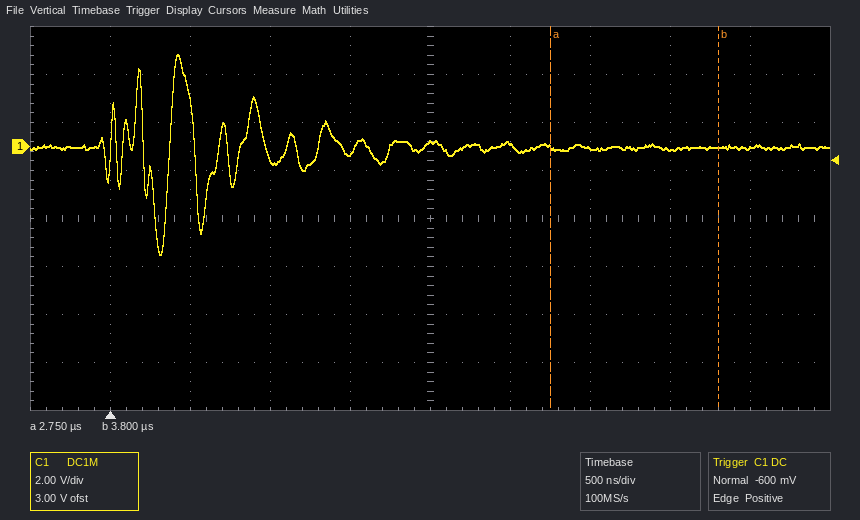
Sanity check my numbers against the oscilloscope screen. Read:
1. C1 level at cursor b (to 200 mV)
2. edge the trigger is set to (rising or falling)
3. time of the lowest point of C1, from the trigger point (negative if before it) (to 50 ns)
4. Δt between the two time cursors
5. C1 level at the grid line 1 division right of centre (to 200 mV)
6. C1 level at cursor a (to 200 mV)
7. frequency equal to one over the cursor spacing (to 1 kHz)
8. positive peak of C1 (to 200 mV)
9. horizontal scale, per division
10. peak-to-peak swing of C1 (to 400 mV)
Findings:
0.0 V
rising
+300 ns
1.05 µs
0.0 V
0.0 V
952 kHz
3.8 V
500 ns
8.4 V
